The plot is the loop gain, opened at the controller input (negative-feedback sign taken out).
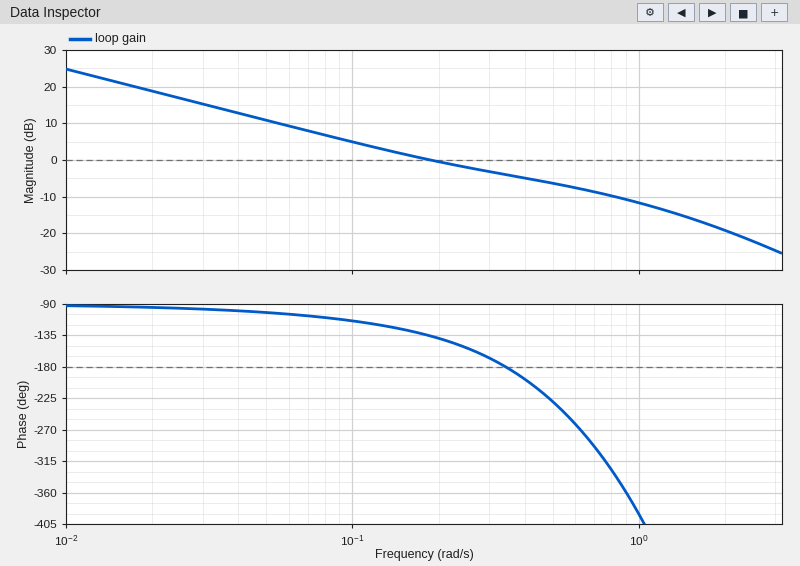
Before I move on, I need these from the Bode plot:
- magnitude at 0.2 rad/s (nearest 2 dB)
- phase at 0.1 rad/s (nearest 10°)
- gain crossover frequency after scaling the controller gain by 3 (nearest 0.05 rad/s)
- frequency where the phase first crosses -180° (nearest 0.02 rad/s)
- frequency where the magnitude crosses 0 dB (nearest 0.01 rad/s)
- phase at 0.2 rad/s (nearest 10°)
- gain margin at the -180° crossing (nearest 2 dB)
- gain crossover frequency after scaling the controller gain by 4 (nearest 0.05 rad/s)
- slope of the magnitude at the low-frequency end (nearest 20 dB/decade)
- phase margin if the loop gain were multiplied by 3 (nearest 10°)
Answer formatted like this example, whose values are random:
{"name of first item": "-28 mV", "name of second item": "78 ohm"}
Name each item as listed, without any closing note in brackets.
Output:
{"magnitude at 0.2 rad/s": "0 dB", "phase at 0.1 rad/s": "-110°", "gain crossover frequency after scaling the controller gain by 3": "0.80 rad/s", "frequency where the phase first crosses -180°": "0.34 rad/s", "frequency where the magnitude crosses 0 dB": "0.19 rad/s", "phase at 0.2 rad/s": "-140°", "gain margin at the -180° crossing": "4 dB", "gain crossover frequency after scaling the controller gain by 4": "1.05 rad/s", "slope of the magnitude at the low-frequency end": "-20 dB/decade", "phase margin if the loop gain were multiplied by 3": "-140°"}
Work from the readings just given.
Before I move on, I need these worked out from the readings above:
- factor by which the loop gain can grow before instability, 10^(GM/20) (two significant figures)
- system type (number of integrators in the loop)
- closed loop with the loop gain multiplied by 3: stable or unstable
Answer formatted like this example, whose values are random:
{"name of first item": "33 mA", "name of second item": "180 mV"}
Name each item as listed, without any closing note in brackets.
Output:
{"factor by which the loop gain can grow before instability, 10^(GM/20)": "1.6", "system type": "1", "closed loop with the loop gain multiplied by 3: stable or unstable": "unstable"}
